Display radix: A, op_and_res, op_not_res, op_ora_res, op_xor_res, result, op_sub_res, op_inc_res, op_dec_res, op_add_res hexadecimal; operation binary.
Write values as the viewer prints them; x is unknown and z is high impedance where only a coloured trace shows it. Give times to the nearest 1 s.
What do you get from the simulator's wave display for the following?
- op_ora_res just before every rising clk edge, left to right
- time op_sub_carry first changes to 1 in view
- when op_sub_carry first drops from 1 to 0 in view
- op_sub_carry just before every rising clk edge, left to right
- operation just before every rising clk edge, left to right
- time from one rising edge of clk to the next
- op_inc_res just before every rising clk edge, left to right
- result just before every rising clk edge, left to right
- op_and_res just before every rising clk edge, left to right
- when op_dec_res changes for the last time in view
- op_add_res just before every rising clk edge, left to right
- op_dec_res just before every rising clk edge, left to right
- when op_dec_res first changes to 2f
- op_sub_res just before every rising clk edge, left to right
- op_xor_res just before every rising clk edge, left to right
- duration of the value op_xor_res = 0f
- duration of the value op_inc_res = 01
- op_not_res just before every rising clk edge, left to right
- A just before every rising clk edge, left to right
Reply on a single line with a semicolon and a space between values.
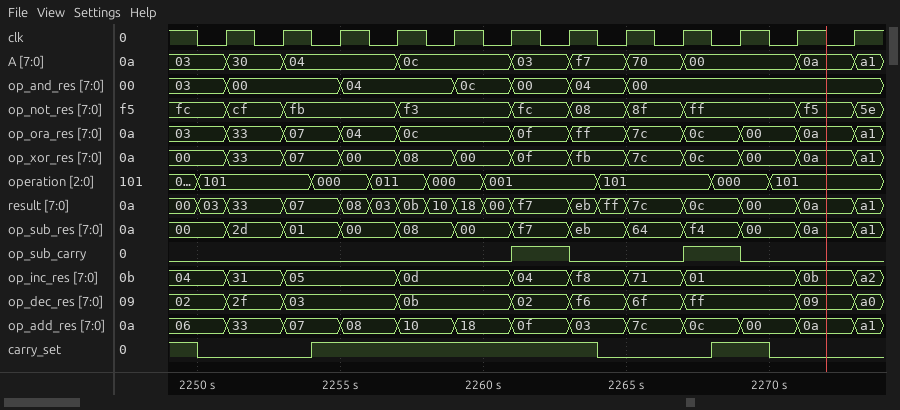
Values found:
03, 33, 07, 04, 0c, 0c, 0f, ff, 7c, 0c, 00, 0a; 2261 s; 2263 s; 0 0 0 0 0 0 1 0 0 1 0 0; 101, 101, 000, 011, 000, 001, 001, 101, 101, 000, 101, 101; 2 s; 04, 31, 05, 05, 0d, 0d, 04, f8, 71, 01, 01, 0b; 03, 33, 07, 03, 10, 00, f7, ff, 7c, 0c, 00, 0a; 03, 00, 00, 04, 04, 0c, 00, 04, 00, 00, 00, 00; 2273 s; 06, 33, 07, 08, 10, 18, 0f, 03, 7c, 0c, 00, 0a; 02, 2f, 03, 03, 0b, 0b, 02, f6, 6f, ff, ff, 09; 2251 s; 00, 2d, 01, 00, 08, 00, f7, eb, 64, f4, 00, 0a; 00, 33, 07, 00, 08, 00, 0f, fb, 7c, 0c, 00, 0a; 2 s; 4 s; fc, cf, fb, fb, f3, f3, fc, 08, 8f, ff, ff, f5; 03, 30, 04, 04, 0c, 0c, 03, f7, 70, 00, 00, 0a
